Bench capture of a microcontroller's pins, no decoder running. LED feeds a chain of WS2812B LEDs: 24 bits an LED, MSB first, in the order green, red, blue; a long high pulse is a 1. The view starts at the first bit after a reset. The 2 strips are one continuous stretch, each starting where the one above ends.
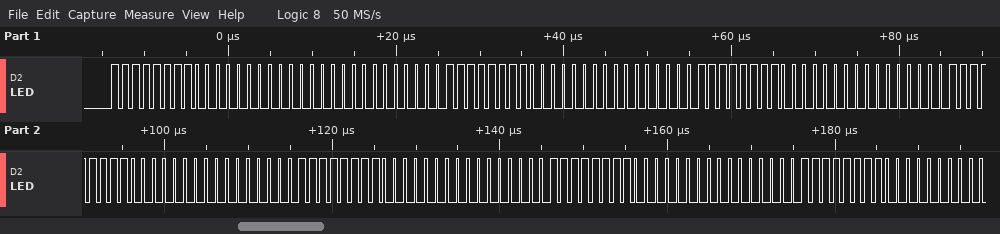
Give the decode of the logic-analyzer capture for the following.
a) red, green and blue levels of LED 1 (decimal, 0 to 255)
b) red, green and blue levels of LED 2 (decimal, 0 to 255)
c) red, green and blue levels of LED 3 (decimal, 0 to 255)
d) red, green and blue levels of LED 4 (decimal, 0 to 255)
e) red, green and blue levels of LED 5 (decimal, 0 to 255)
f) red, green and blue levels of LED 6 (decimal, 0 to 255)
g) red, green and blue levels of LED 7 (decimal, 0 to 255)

0, 255, 0
255, 0, 0
255, 0, 0
255, 0, 0
255, 0, 0
255, 0, 0
255, 0, 0
